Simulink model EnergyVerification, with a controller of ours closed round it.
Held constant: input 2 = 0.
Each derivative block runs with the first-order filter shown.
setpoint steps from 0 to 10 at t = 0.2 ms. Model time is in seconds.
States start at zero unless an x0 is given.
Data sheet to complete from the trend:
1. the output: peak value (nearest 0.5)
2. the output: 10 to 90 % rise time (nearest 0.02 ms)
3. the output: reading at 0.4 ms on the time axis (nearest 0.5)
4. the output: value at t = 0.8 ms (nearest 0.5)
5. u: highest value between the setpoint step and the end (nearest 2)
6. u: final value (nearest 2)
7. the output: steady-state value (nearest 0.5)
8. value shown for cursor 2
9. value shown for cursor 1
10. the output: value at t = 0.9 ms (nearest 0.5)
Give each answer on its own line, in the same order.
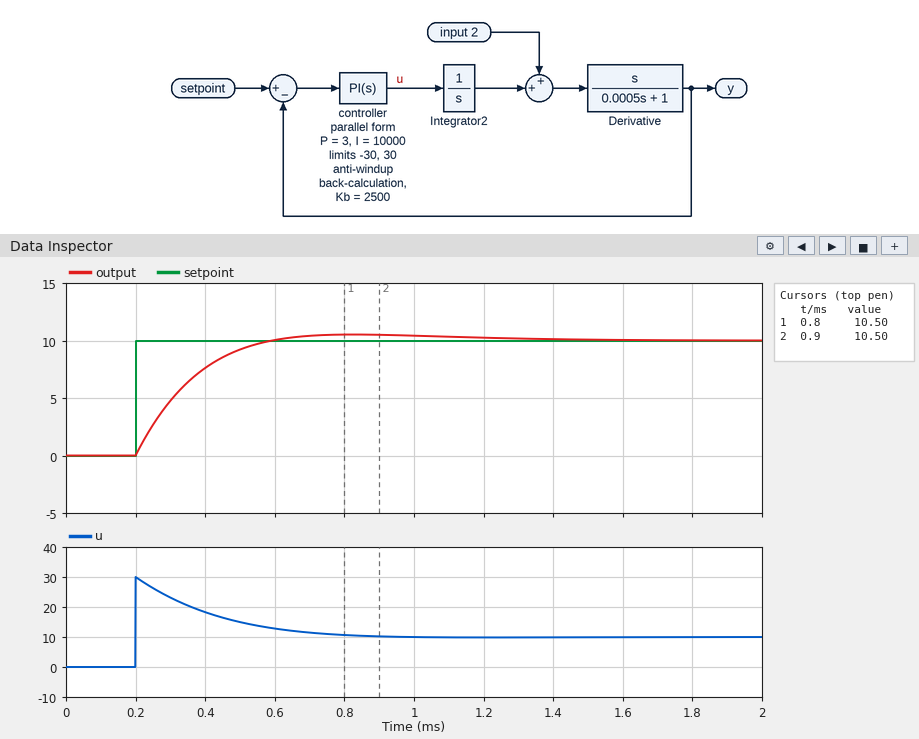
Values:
10.5
0.26 ms
7.5
10.5
30
10
10.0
10.50
10.50
10.5
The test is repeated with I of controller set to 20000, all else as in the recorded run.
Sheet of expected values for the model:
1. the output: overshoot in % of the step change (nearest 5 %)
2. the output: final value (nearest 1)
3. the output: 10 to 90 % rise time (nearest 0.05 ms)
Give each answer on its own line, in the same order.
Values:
15 %
10
0.20 ms
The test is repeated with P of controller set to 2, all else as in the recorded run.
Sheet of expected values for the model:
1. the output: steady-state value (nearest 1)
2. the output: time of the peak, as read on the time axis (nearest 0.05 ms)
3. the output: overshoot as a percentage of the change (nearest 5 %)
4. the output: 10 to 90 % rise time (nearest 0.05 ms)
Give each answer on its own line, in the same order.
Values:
10
0.85 ms
10 %
0.30 ms
